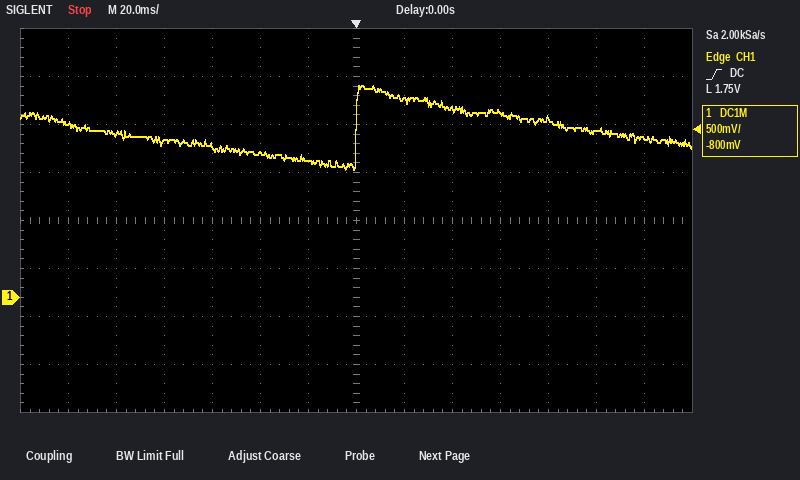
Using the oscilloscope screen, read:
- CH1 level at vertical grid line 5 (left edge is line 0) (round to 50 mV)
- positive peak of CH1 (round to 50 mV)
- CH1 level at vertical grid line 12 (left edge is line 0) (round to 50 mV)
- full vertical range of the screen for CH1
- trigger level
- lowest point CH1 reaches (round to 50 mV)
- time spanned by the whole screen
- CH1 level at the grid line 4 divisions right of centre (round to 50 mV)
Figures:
1.50 V
2.20 V
1.75 V
4 V
1.75 V
1.35 V
280 ms
1.85 V
